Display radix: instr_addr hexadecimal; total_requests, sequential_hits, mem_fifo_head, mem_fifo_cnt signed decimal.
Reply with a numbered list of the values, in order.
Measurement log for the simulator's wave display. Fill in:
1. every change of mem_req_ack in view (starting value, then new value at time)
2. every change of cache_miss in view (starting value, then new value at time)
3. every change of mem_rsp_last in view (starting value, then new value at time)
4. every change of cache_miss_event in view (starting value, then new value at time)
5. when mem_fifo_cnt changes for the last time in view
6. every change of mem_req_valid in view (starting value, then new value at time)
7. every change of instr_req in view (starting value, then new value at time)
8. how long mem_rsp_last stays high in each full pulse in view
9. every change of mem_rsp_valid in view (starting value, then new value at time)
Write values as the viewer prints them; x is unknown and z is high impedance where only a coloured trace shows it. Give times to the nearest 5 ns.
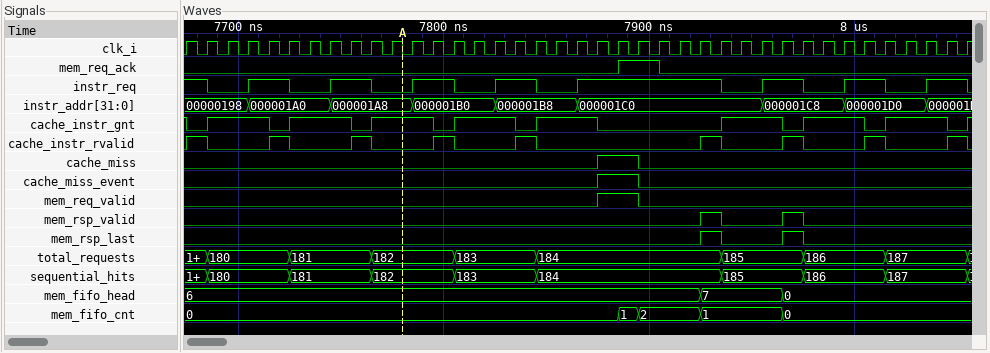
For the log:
1. 0, 1 at 7885 ns, 0 at 7905 ns
2. 0, 1 at 7875 ns, 0 at 7895 ns
3. 0, 1 at 7925 ns, 0 at 7935 ns, 1 at 7965 ns, 0 at 7975 ns
4. 0, 1 at 7875 ns, 0 at 7895 ns
5. 7965 ns
6. 0, 1 at 7875 ns, 0 at 7895 ns
7. 1, 0 at 7685 ns, 1 at 7705 ns, 0 at 7725 ns, 1 at 7745 ns, 0 at 7765 ns, 1 at 7785 ns, 0 at 7805 ns, 1 at 7825 ns, 0 at 7845 ns, 1 at 7865 ns, 0 at 7935 ns, 1 at 7955 ns, 0 at 7975 ns, 1 at 7995 ns, 0 at 8015 ns, 1 at 8035 ns, 0 at 8055 ns
8. 10 ns, 10 ns
9. 0, 1 at 7925 ns, 0 at 7935 ns, 1 at 7965 ns, 0 at 7975 ns
